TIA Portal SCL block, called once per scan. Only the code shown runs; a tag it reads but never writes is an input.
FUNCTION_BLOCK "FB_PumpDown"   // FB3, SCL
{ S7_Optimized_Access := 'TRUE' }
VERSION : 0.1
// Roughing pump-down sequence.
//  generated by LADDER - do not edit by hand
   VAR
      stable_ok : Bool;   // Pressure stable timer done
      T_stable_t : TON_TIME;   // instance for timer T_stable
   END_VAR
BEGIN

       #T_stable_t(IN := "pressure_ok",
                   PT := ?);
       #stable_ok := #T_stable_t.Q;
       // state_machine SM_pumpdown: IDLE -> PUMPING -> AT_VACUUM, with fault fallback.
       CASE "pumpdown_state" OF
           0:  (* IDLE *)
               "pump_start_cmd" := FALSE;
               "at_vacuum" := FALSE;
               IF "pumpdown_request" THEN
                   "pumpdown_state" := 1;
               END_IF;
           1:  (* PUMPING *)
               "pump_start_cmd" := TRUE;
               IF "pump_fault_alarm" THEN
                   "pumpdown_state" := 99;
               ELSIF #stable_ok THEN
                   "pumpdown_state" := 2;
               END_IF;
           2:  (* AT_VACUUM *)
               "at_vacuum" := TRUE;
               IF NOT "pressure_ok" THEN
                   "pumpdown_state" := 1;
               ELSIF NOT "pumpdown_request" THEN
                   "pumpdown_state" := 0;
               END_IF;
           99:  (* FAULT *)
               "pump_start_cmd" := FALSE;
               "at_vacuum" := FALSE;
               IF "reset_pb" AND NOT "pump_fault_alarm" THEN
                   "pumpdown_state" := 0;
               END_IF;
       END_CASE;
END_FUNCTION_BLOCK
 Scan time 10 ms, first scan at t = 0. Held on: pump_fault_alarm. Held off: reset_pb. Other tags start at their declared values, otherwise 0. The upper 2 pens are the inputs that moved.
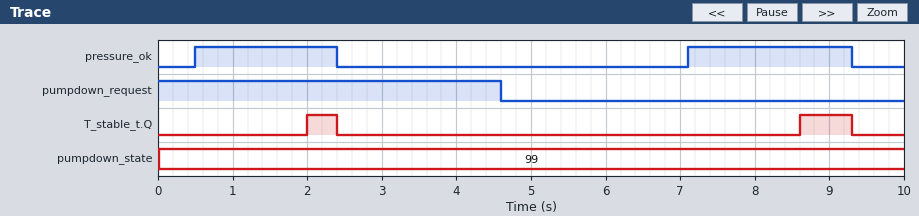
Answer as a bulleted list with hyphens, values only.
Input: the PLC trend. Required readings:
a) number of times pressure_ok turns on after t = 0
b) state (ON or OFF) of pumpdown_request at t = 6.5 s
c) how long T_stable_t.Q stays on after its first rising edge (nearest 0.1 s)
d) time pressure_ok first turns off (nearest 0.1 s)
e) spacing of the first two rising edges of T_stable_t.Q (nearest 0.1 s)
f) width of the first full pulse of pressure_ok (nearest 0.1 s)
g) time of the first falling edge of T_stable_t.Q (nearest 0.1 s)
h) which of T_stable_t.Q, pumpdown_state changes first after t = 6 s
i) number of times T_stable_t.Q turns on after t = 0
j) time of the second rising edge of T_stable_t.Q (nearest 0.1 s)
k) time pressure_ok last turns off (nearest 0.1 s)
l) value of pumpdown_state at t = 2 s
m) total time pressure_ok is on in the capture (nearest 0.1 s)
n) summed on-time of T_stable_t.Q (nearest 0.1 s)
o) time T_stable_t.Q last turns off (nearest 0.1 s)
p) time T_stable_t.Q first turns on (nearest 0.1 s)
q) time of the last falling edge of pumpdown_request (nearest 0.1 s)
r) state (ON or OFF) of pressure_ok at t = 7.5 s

- 2
- OFF
- 0.4 s
- 2.4 s
- 6.6 s
- 1.9 s
- 2.4 s
- T_stable_t.Q
- 2
- 8.6 s
- 9.3 s
- 99
- 4.1 s
- 1.1 s
- 9.3 s
- 2.0 s
- 4.6 s
- ON
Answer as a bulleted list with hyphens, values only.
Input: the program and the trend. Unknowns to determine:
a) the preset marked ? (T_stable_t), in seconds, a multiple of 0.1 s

- 1.5 s
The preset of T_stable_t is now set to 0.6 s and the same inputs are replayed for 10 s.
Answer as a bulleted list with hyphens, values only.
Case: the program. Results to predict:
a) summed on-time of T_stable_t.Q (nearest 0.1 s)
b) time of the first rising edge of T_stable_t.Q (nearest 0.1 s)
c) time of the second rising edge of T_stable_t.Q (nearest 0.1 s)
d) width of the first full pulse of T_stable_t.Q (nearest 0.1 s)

- 2.9 s
- 1.1 s
- 7.7 s
- 1.3 s
